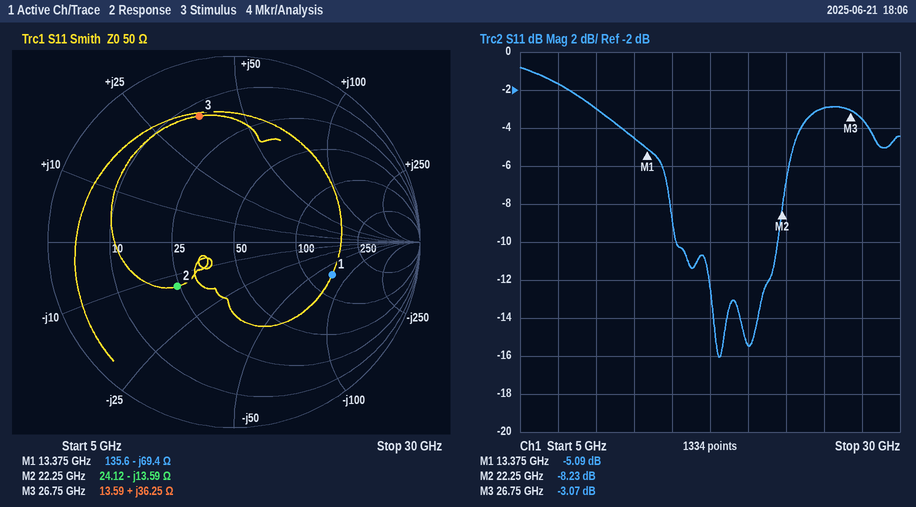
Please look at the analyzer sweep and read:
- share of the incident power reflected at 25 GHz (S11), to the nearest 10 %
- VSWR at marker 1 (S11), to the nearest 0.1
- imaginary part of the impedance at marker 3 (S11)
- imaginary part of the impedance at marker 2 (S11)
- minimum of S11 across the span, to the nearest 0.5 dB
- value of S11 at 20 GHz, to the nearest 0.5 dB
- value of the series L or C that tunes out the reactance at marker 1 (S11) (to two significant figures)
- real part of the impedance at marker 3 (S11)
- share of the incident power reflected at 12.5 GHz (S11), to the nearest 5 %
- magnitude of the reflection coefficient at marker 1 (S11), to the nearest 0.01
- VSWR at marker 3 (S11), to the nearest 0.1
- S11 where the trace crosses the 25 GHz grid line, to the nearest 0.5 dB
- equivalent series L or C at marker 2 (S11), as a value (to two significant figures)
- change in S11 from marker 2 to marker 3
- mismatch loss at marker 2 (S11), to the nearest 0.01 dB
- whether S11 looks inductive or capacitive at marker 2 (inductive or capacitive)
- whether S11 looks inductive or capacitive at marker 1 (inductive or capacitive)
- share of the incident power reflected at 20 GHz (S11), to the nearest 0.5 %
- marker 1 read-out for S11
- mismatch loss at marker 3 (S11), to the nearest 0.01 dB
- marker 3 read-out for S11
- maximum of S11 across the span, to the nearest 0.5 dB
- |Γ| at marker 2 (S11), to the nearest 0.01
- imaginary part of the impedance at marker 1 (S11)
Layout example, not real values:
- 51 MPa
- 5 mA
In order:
- 50 %
- 3.5
- +36.25 Ω
- -13.59 Ω
- -16.0 dB
- -15.5 dB
- 830 pH
- 13.59 Ω
- 35 %
- 0.56
- 5.7
- -3.0 dB
- 530 fF
- 5.16 dB
- 0.71 dB
- capacitive
- capacitive
- 3.0 %
- -5.09 dB
- 2.95 dB
- -3.07 dB
- -1.0 dB
- 0.39
- -69.4 Ω
